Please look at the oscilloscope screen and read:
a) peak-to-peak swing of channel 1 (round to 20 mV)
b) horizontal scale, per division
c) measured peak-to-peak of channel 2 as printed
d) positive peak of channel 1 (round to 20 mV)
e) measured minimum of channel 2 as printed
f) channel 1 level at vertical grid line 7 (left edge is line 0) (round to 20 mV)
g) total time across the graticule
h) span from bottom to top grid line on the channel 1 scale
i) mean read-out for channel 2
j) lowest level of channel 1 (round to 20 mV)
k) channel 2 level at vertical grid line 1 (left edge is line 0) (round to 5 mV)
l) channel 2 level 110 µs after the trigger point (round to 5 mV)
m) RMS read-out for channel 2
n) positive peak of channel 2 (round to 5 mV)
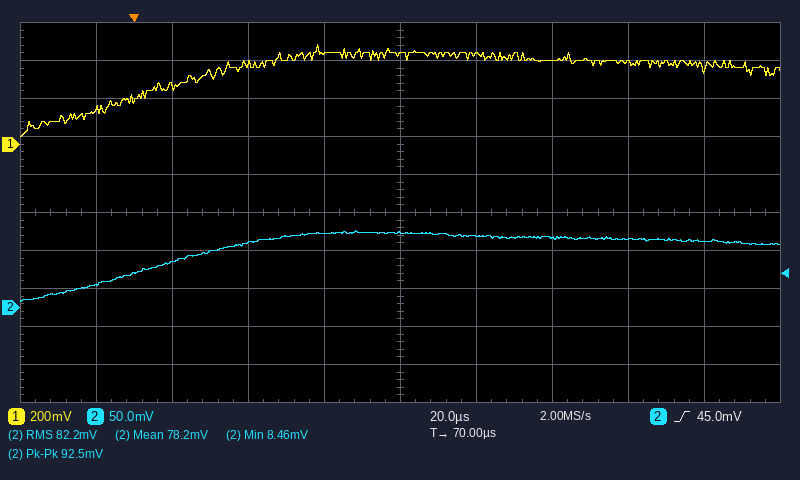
480 mV
20 µs
92.5 mV
520 mV
8.46 mV
440 mV
200 µs
2 V
78.2 mV
40 mV
30 mV
90 mV
82.2 mV
100 mV
